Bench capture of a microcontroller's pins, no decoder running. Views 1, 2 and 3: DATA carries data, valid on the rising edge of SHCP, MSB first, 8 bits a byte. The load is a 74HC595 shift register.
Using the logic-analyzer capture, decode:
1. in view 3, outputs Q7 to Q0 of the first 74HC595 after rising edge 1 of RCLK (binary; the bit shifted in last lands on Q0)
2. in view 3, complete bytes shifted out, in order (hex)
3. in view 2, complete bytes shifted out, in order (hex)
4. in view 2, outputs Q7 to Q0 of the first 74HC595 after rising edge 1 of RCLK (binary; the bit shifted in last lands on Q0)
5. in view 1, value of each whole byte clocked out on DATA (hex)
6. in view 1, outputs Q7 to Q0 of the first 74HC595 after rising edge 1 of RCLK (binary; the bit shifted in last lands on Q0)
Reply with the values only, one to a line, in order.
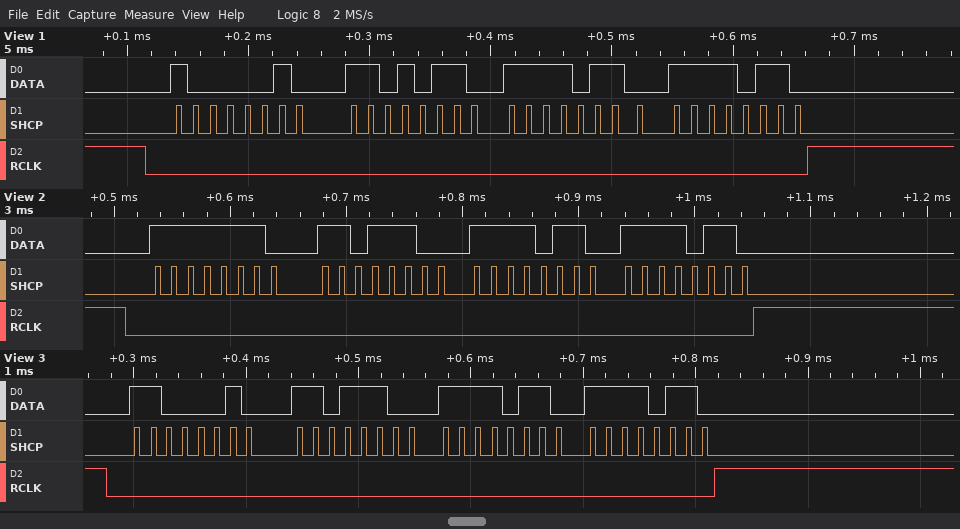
11110110
C2 DC F6 F6
FE DC F6 F6
11110110
82 D6 F6 F6
11110110
